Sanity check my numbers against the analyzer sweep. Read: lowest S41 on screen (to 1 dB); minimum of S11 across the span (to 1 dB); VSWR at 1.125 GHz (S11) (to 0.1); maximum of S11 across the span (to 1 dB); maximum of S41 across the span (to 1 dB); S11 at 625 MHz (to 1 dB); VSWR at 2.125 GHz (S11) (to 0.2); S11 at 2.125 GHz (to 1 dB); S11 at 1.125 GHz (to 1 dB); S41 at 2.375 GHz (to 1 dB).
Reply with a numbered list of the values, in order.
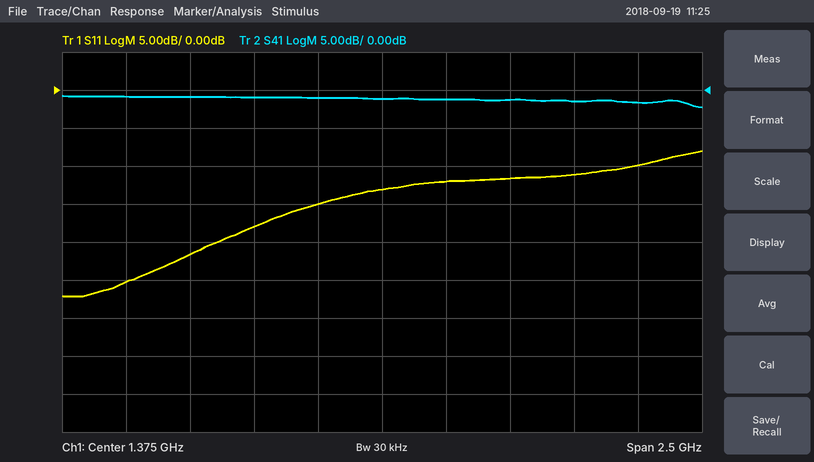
1. -2 dB
2. -27 dB
3. 1.4
4. -8 dB
5. -1 dB
6. -22 dB
7. 1.8
8. -11 dB
9. -15 dB
10. -2 dB
